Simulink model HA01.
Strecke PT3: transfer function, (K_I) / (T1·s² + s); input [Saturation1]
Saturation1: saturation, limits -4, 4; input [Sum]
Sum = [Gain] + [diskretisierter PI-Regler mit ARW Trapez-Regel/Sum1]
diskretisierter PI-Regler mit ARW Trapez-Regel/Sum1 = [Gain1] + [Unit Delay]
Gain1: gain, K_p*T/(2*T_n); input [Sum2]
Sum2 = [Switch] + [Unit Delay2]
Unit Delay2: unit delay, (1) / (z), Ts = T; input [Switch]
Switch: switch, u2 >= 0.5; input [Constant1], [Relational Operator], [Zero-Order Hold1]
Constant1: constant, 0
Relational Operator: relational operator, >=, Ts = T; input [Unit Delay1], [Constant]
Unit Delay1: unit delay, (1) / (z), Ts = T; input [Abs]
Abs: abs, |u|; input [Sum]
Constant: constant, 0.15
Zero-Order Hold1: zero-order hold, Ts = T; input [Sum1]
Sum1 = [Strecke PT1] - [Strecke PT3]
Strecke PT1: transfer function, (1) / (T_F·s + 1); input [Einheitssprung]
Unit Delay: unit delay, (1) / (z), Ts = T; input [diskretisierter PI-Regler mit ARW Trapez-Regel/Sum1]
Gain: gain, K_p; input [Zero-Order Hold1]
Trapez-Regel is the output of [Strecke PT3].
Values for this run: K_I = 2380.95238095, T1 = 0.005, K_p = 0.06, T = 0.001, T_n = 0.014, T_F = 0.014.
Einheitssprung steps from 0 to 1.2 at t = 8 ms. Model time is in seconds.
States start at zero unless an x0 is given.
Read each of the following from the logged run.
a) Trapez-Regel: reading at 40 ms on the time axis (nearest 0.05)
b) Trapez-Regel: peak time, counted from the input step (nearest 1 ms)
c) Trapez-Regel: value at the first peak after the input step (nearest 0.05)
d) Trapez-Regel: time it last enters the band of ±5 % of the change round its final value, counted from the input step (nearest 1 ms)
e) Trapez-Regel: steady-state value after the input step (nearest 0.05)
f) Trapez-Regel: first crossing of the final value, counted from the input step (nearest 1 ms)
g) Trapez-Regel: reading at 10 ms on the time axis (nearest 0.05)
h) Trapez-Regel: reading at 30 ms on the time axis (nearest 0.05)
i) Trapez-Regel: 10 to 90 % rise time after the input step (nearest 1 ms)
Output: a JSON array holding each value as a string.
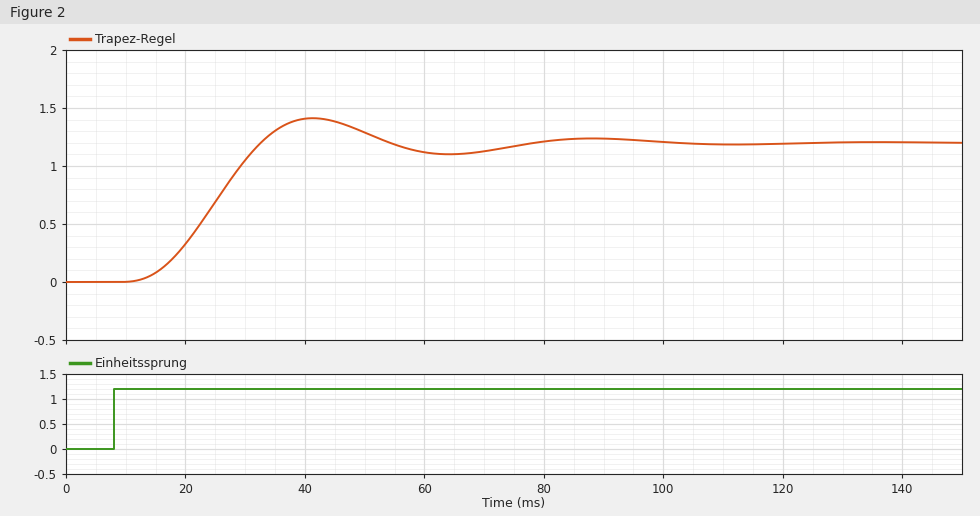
["1.40", "33 ms", "1.40", "64 ms", "1.20", "25 ms", "0.00", "1.05", "14 ms"]
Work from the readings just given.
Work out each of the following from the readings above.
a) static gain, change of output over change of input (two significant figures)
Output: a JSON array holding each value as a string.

["1.0"]
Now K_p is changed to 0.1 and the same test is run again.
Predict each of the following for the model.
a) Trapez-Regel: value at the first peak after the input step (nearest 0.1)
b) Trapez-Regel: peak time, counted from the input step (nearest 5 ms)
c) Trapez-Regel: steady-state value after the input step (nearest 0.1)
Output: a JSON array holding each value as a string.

["1.3", "25 ms", "1.2"]
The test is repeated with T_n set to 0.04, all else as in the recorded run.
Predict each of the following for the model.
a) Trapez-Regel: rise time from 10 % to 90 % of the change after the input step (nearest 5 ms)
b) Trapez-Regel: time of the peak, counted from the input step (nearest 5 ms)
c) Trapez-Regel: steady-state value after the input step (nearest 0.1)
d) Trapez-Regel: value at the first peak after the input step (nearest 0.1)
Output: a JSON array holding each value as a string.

["20 ms", "40 ms", "1.2", "1.3"]
